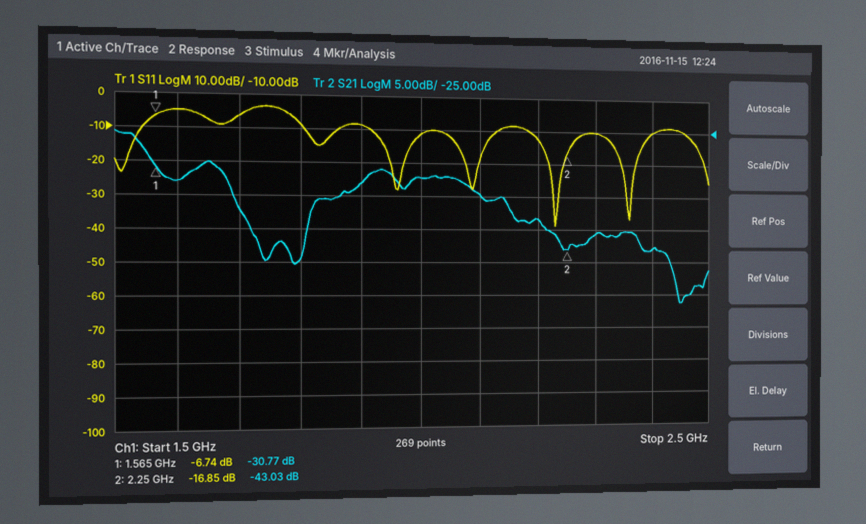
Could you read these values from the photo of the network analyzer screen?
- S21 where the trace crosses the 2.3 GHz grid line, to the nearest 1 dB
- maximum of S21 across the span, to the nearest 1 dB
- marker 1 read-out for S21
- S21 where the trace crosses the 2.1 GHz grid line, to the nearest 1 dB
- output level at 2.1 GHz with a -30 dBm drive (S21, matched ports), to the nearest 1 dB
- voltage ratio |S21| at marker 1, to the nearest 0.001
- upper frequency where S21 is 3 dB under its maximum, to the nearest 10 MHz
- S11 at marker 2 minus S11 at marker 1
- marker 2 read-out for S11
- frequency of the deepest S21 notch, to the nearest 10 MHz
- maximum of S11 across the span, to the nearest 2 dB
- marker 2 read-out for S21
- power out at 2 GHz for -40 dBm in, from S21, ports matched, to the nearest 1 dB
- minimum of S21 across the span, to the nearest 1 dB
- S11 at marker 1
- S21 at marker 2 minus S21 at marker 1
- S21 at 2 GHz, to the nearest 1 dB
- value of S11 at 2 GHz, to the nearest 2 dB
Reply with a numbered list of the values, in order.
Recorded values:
1. -41 dB
2. -26 dB
3. -30.77 dB
4. -35 dB
5. -65 dBm
6. 0.029
7. 1.55 GHz
8. -10.11 dB
9. -16.85 dB
10. 2.45 GHz
11. -4 dB
12. -43.03 dB
13. -72 dBm
14. -51 dB
15. -6.74 dB
16. -12.26 dB
17. -32 dB
18. -12 dB
